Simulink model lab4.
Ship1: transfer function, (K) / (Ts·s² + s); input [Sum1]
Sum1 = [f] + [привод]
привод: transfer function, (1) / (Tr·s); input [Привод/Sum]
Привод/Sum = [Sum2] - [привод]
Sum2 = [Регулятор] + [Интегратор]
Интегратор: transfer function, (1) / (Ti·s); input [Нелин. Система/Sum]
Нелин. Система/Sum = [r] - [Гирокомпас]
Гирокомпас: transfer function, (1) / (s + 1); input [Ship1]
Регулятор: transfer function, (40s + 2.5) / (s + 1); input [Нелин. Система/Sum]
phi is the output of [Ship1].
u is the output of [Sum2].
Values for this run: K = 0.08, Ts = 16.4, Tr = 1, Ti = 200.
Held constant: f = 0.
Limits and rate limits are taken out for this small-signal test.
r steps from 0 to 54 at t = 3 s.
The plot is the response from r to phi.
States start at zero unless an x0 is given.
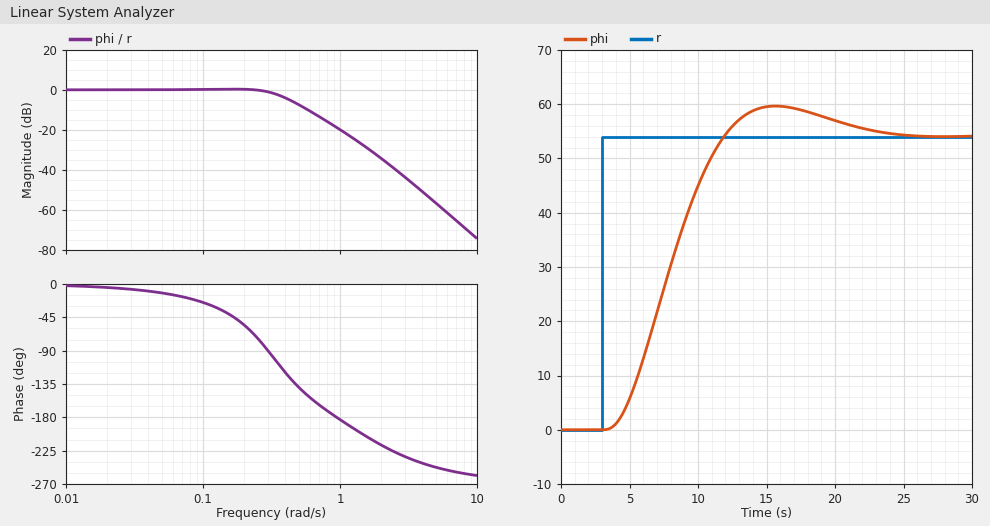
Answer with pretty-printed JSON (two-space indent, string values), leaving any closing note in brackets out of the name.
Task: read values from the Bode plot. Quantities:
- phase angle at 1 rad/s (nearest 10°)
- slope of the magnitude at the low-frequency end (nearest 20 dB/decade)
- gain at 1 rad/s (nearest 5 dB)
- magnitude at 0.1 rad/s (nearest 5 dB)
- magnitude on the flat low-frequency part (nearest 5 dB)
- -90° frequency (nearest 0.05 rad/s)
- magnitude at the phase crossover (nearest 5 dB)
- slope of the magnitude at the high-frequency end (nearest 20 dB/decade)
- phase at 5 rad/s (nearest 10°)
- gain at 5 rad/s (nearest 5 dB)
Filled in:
{
  "phase angle at 1 rad/s": "-180°",
  "slope of the magnitude at the low-frequency end": "0 dB/decade",
  "gain at 1 rad/s": "-20 dB",
  "magnitude at 0.1 rad/s": "0 dB",
  "magnitude on the flat low-frequency part": "0 dB",
  "-90° frequency": "0.30 rad/s",
  "magnitude at the phase crossover": "-20 dB",
  "slope of the magnitude at the high-frequency end": "-60 dB/decade",
  "phase at 5 rad/s": "-250°",
  "gain at 5 rad/s": "-55 dB"
}
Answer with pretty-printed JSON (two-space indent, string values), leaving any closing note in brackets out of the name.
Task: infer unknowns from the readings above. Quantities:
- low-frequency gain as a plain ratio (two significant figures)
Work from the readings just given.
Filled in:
{
  "low-frequency gain as a plain ratio": "1.0"
}
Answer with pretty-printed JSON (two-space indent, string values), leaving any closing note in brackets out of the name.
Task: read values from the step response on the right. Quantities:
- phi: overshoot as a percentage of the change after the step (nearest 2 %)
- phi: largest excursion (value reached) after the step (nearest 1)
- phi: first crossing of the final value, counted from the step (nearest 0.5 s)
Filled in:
{
  "phi: overshoot as a percentage of the change after the step": "10 %",
  "phi: largest excursion (value reached) after the step": "60",
  "phi: first crossing of the final value, counted from the step": "9.0 s"
}
